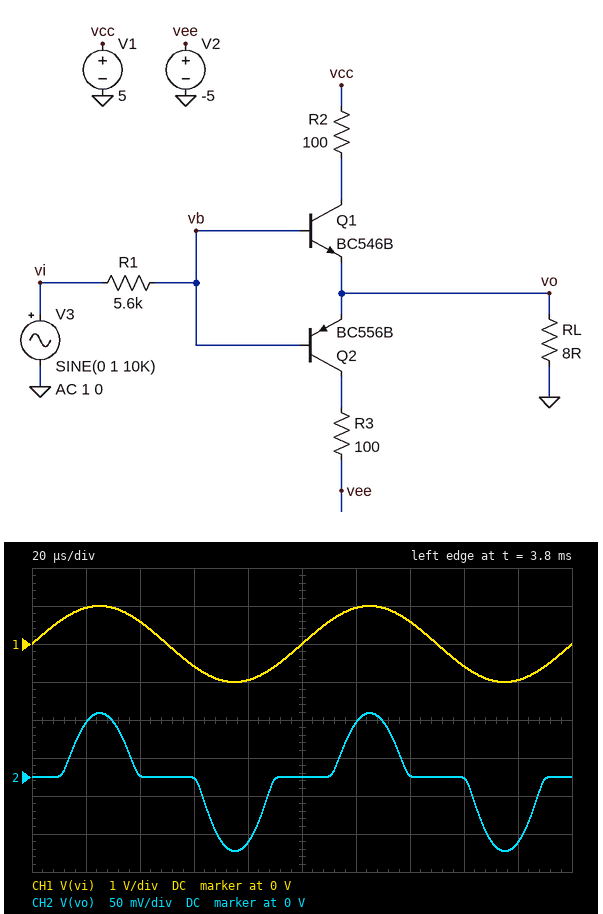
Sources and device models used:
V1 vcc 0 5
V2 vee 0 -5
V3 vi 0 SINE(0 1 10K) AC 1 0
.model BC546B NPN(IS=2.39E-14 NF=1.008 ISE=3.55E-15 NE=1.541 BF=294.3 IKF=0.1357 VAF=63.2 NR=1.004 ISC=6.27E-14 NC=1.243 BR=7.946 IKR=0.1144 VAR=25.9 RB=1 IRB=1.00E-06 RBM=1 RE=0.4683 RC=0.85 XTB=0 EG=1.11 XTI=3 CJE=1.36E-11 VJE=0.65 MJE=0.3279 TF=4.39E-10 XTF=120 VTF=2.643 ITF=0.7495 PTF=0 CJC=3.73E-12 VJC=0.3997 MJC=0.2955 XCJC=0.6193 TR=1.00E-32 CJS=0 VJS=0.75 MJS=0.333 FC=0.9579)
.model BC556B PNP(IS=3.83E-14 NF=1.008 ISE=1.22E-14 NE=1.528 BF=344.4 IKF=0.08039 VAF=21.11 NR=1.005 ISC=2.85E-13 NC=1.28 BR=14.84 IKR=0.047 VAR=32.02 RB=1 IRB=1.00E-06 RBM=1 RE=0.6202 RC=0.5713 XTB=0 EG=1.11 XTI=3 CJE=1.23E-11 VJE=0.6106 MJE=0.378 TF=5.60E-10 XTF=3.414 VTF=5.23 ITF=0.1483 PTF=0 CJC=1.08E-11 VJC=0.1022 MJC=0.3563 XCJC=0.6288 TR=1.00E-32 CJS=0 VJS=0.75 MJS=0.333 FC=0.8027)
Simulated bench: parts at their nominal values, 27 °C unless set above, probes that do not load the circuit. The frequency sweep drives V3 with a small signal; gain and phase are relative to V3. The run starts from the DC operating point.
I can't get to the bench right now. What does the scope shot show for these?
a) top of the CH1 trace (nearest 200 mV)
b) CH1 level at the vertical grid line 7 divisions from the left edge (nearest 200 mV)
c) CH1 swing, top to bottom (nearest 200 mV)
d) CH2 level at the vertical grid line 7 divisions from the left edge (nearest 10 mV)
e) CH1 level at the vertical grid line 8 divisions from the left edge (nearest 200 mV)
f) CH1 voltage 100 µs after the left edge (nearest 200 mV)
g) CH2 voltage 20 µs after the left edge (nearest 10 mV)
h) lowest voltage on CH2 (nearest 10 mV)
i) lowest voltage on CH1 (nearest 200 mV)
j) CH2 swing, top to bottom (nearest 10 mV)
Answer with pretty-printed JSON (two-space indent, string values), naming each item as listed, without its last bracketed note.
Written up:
{
  "top of the CH1 trace": "1.0 V",
  "CH1 level at the vertical grid line 7 divisions from the left edge": "600 mV",
  "CH1 swing, top to bottom": "2.0 V",
  "CH2 level at the vertical grid line 7 divisions from the left edge": "0 V",
  "CH1 level at the vertical grid line 8 divisions from the left edge": "-600 mV",
  "CH1 voltage 100 µs after the left edge": "0 V",
  "CH2 voltage 20 µs after the left edge": "70 mV",
  "lowest voltage on CH2": "-100 mV",
  "lowest voltage on CH1": "-1.0 V",
  "CH2 swing, top to bottom": "180 mV"
}
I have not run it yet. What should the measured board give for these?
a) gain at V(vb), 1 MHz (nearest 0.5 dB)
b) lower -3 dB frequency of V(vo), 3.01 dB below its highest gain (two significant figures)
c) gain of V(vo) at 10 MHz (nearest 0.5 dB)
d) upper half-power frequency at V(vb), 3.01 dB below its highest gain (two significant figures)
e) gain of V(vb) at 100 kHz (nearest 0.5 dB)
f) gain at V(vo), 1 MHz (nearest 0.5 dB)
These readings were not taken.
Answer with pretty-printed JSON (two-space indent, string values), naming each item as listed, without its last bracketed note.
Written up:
{
  "gain at V(vb), 1 MHz": "-3.5 dB",
  "lower -3 dB frequency of V(vo), 3.01 dB below its highest gain": "940 kHz",
  "gain of V(vo) at 10 MHz": "-58.5 dB",
  "upper half-power frequency at V(vb), 3.01 dB below its highest gain": "940 kHz",
  "gain of V(vb) at 100 kHz": "0 dB",
  "gain at V(vo), 1 MHz": "-61.0 dB"
}
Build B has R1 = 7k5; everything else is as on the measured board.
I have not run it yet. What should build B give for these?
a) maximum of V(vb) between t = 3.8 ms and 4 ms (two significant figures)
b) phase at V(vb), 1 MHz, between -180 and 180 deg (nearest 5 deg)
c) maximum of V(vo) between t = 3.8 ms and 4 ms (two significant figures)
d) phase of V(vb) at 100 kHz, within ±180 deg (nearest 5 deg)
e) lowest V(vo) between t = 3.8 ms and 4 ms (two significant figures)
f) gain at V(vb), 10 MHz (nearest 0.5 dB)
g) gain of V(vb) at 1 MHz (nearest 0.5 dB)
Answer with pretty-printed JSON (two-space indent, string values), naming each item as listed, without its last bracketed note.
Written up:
{
  "maximum of V(vb) between t = 3.8 ms and 4 ms": "770 mV",
  "phase at V(vb), 1 MHz, between -180 and 180 deg": "-55 deg",
  "maximum of V(vo) between t = 3.8 ms and 4 ms": "70 mV",
  "phase of V(vb) at 100 kHz, within ±180 deg": "-10 deg",
  "lowest V(vo) between t = 3.8 ms and 4 ms": "-83 mV",
  "gain at V(vb), 10 MHz": "-23.0 dB",
  "gain of V(vb) at 1 MHz": "-5.0 dB"
}
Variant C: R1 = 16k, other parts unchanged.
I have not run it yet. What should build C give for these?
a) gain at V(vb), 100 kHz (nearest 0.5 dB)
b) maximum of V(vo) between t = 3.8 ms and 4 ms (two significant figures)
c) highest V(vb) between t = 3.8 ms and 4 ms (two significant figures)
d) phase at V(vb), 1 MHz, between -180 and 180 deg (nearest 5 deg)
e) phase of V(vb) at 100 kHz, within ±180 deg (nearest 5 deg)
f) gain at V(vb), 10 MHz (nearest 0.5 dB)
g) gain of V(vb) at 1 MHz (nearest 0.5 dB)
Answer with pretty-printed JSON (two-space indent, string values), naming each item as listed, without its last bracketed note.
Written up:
{
  "gain at V(vb), 100 kHz": "-0.5 dB",
  "maximum of V(vo) between t = 3.8 ms and 4 ms": "41 mV",
  "highest V(vb) between t = 3.8 ms and 4 ms": "720 mV",
  "phase at V(vb), 1 MHz, between -180 and 180 deg": "-70 deg",
  "phase of V(vb) at 100 kHz, within ±180 deg": "-15 deg",
  "gain at V(vb), 10 MHz": "-29.5 dB",
  "gain of V(vb) at 1 MHz": "-10.0 dB"
}
